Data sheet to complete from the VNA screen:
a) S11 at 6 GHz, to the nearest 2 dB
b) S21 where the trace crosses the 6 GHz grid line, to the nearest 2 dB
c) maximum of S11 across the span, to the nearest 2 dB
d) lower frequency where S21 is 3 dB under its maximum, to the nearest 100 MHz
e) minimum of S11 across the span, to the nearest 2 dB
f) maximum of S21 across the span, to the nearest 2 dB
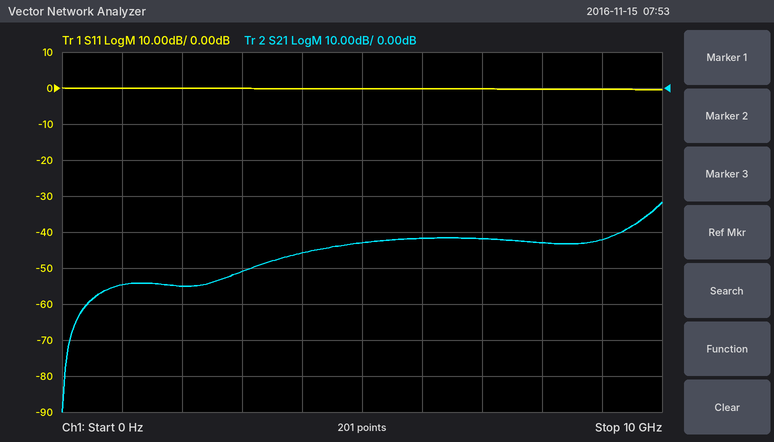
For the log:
0 dB
-42 dB
0 dB
9.8 GHz
0 dB
-32 dB
